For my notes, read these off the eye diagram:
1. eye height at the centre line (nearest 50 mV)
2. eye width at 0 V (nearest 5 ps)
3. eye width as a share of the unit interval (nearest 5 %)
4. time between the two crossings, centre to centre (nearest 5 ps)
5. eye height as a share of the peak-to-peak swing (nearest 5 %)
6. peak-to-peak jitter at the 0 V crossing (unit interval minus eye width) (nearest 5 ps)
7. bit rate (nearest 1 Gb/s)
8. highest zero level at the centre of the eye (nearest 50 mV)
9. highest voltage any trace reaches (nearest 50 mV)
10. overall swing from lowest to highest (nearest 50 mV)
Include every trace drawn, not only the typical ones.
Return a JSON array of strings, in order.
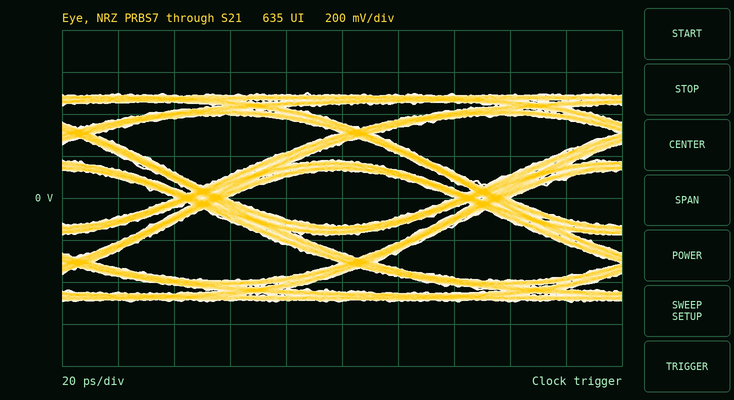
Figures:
["250 mV", "80 ps", "80 %", "100 ps", "25 %", "20 ps", "10 Gb/s", "-150 mV", "500 mV", "1.00 V"]
